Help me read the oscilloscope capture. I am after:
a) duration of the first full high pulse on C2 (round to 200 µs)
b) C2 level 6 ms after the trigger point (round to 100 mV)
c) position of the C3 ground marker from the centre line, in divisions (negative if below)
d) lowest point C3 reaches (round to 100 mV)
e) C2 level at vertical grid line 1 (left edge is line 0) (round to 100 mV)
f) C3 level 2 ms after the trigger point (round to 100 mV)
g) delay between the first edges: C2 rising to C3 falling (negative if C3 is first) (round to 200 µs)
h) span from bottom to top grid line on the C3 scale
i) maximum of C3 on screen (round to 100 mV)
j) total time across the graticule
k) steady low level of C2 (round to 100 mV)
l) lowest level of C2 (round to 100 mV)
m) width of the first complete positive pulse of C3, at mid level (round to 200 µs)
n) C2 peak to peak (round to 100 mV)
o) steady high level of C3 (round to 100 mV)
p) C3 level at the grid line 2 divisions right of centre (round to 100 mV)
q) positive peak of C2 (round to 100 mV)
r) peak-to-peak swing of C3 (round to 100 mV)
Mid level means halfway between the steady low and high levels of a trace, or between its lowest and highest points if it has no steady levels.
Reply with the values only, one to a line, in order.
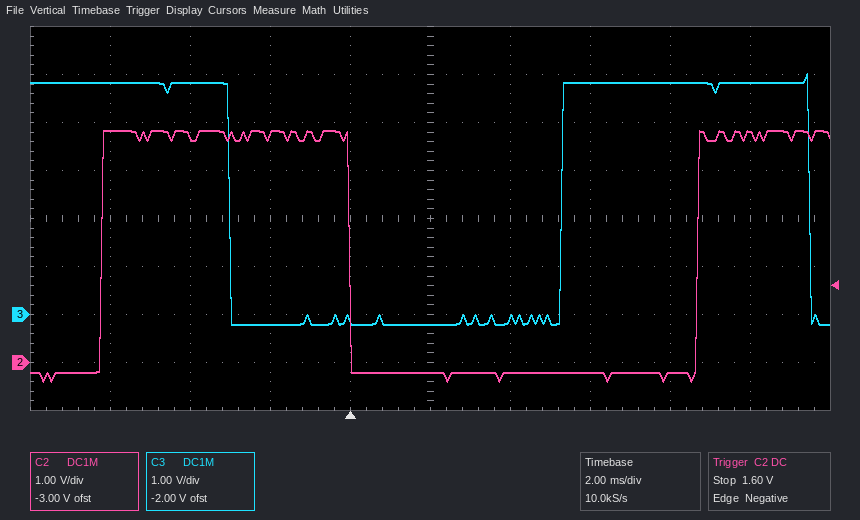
6.2 ms
-200 mV
-2.0 div
-200 mV
4.8 V
-200 mV
+3.2 ms
8 V
5.0 V
20 ms
-200 mV
-400 mV
6.2 ms
5.2 V
4.8 V
4.8 V
4.8 V
5.2 V
